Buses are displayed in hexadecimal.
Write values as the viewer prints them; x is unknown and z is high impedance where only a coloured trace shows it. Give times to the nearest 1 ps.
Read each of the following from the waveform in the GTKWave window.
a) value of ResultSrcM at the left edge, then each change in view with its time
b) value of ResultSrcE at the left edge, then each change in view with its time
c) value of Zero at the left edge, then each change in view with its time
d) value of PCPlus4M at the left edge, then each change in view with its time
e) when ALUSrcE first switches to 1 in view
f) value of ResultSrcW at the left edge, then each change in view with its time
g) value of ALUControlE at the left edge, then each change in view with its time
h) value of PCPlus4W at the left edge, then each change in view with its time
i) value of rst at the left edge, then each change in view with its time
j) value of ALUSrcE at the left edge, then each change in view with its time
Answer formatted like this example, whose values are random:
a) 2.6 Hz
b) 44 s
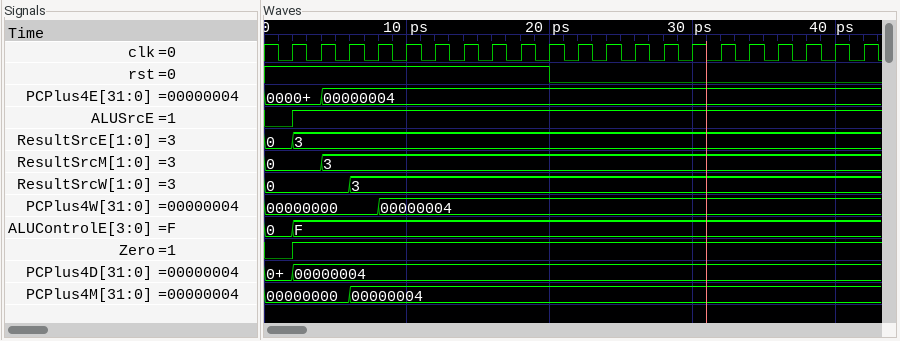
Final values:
a) 0, 3 at 4 ps
b) 0, 3 at 2 ps
c) 0, 1 at 2 ps
d) 00000000, 00000004 at 6 ps
e) 2 ps
f) 0, 3 at 6 ps
g) 0, F at 2 ps
h) 00000000, 00000004 at 8 ps
i) 1, 0 at 20 ps
j) 0, 1 at 2 ps
